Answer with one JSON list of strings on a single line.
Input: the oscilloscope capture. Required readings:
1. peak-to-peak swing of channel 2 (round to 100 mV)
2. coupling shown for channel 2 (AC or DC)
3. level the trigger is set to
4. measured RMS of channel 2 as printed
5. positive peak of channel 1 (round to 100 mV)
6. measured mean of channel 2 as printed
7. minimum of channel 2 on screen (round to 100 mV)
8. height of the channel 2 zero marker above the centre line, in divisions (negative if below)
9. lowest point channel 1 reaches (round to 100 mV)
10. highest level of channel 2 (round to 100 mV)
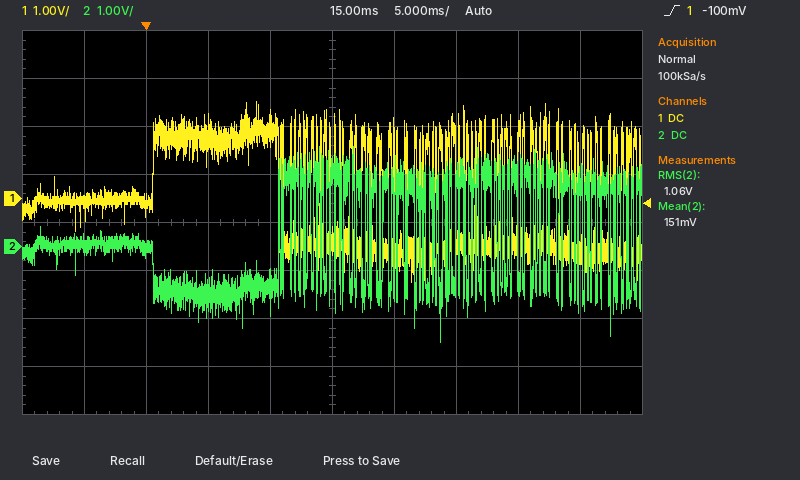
["4.1 V", "DC", "-100 mV", "1.06 V", "2.0 V", "151 mV", "-2.0 V", "-0.5 div", "-1.7 V", "2.1 V"]
